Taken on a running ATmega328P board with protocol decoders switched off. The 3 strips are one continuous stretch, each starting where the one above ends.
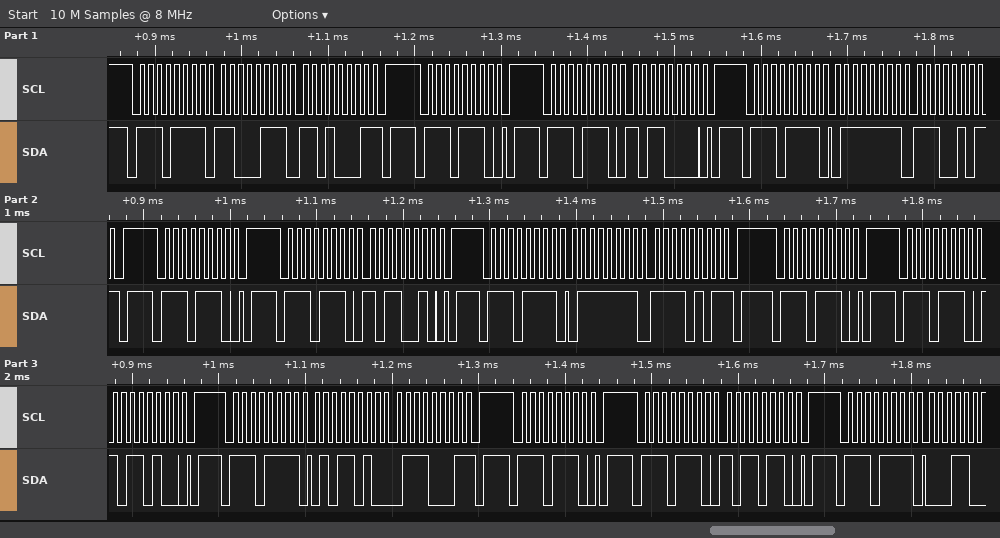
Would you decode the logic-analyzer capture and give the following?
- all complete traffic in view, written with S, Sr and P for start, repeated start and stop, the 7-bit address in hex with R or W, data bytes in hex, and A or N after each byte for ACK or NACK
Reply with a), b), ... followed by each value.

a) S 77R A C7 A D1 N P S 77W A P S 77W A B0 A P S 77R A 7F A E5 N P S 77W A P S 77W A B2 A P S 77R A 7F A F5 N P S 77W A P S 77W A B4 A P S 77R A 5A A 71 N P S 77W A P S 77W A B6 A P S 77R A
